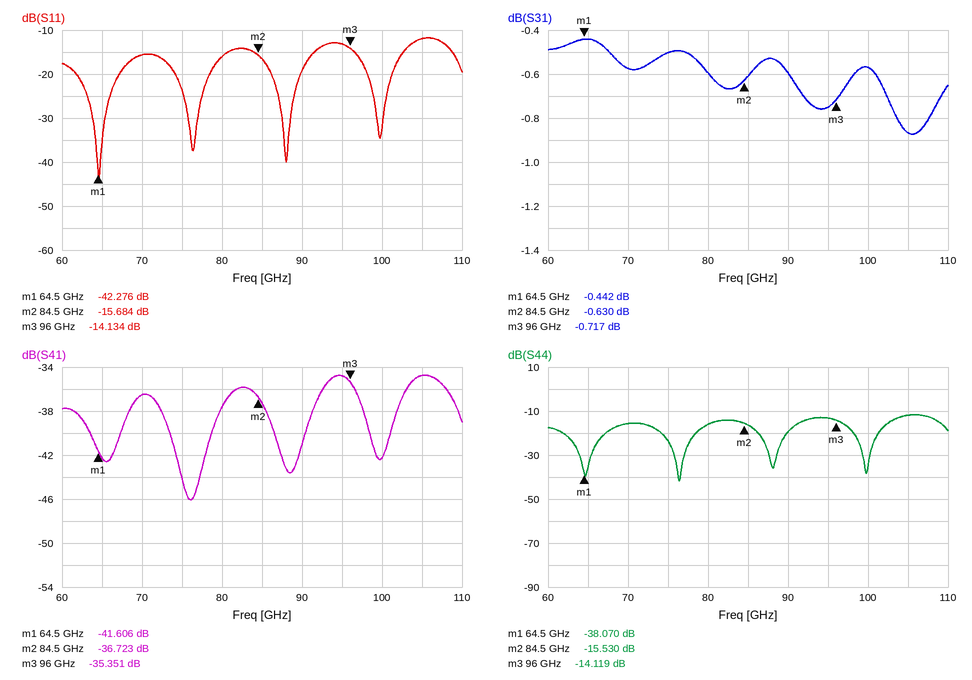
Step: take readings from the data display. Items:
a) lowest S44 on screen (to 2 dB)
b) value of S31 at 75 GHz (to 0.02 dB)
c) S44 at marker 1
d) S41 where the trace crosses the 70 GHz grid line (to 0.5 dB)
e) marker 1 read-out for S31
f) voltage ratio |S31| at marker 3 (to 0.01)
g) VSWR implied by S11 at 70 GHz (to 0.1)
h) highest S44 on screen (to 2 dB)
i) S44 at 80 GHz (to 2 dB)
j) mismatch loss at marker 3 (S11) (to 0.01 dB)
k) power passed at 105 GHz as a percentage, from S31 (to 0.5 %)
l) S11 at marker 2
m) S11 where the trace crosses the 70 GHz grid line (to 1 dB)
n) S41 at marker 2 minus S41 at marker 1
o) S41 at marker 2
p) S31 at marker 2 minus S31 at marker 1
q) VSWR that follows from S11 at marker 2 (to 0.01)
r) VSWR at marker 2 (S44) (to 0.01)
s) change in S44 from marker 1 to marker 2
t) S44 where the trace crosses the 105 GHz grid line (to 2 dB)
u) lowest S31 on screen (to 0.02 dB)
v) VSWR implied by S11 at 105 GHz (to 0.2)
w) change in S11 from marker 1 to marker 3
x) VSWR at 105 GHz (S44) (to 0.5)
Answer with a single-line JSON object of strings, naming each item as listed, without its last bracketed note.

{"lowest S44 on screen": "-42 dB", "value of S31 at 75 GHz": "-0.50 dB", "S44 at marker 1": "-38.070 dB", "S41 where the trace crosses the 70 GHz grid line": "-36.5 dB", "marker 1 read-out for S31": "-0.442 dB", "voltage ratio |S31| at marker 3": "0.92", "VSWR implied by S11 at 70 GHz": "1.4", "highest S44 on screen": "-12 dB", "S44 at 80 GHz": "-16 dB", "mismatch loss at marker 3 (S11)": "0.17 dB", "power passed at 105 GHz as a percentage, from S31": "82.0 %", "S11 at marker 2": "-15.684 dB", "S11 where the trace crosses the 70 GHz grid line": "-16 dB", "S41 at marker 2 minus S41 at marker 1": "4.883 dB", "S41 at marker 2": "-36.723 dB", "S31 at marker 2 minus S31 at marker 1": "-0.188 dB", "VSWR that follows from S11 at marker 2": "1.39", "VSWR at marker 2 (S44)": "1.40", "change in S44 from marker 1 to marker 2": "22.540 dB", "S44 where the trace crosses the 105 GHz grid line": "-12 dB", "lowest S31 on screen": "-0.88 dB", "VSWR implied by S11 at 105 GHz": "1.6", "change in S11 from marker 1 to marker 3": "28.142 dB", "VSWR at 105 GHz (S44)": "1.5"}
